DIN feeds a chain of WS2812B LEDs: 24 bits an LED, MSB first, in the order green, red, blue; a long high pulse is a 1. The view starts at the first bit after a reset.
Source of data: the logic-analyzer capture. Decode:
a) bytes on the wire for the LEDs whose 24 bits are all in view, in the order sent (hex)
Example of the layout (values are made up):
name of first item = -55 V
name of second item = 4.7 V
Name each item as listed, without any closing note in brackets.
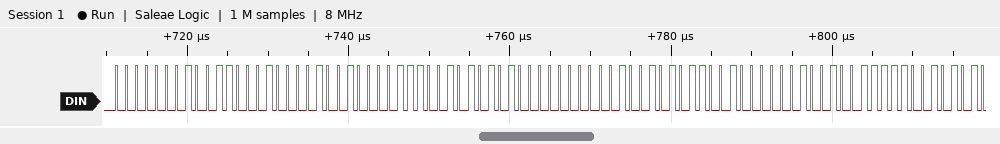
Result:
bytes on the wire for the LEDs whose 24 bits are all in view, in the order sent = 01 31 09 0E 55 00 25 64 09
